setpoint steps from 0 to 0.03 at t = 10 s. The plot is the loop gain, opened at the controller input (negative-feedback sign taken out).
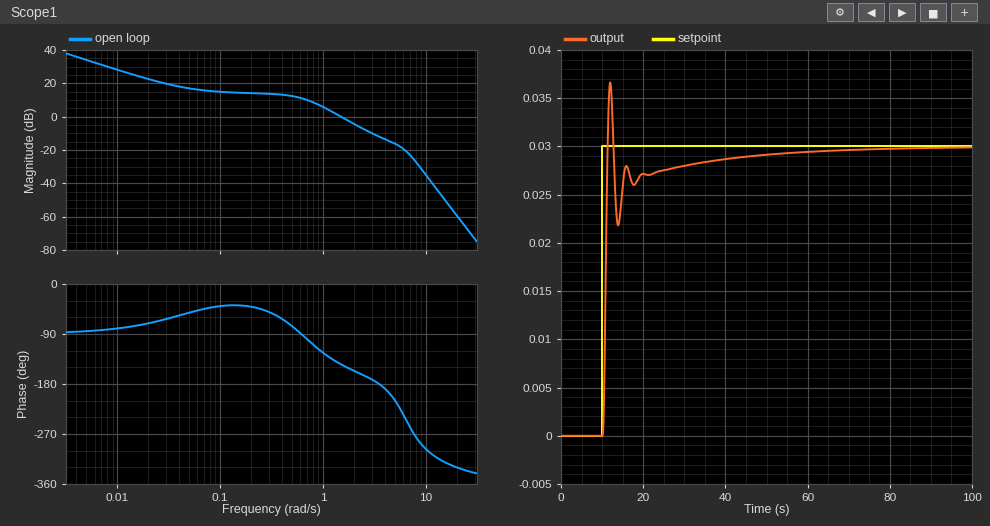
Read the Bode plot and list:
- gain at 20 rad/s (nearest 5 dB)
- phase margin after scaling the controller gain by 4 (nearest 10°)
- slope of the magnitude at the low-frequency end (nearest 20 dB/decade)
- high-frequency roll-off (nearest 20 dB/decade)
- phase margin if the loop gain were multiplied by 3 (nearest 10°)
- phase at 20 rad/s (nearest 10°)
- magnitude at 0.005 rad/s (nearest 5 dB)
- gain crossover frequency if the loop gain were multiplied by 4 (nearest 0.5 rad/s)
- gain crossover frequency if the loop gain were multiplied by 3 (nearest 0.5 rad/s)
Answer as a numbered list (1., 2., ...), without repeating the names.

1. -60 dB
2. 0°
3. -20 dB/decade
4. -80 dB/decade
5. 10°
6. -330°
7. 35 dB
8. 3.5 rad/s
9. 3.0 rad/s
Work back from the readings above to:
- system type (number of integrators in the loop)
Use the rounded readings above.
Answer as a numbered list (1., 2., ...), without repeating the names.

1. 1
